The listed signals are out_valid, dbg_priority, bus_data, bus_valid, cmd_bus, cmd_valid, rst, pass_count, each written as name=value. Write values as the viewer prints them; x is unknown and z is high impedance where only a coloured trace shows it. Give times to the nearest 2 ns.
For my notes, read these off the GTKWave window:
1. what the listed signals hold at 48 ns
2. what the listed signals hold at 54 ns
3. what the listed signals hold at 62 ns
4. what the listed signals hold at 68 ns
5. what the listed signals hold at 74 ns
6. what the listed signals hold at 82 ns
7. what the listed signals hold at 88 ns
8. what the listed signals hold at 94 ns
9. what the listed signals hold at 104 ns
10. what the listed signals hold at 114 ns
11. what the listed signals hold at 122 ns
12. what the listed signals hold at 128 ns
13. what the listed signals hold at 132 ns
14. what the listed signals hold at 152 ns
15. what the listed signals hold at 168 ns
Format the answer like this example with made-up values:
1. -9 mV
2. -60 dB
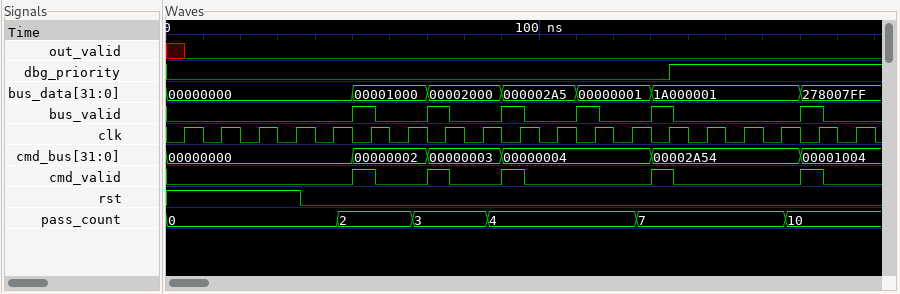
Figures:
1. out_valid=0, dbg_priority=0, bus_data=00000000, bus_valid=0, cmd_bus=00000000, cmd_valid=0, rst=0, pass_count=2
2. out_valid=0, dbg_priority=0, bus_data=00001000, bus_valid=1, cmd_bus=00000002, cmd_valid=1, rst=0, pass_count=2
3. out_valid=0, dbg_priority=0, bus_data=00001000, bus_valid=0, cmd_bus=00000002, cmd_valid=0, rst=0, pass_count=2
4. out_valid=0, dbg_priority=0, bus_data=00001000, bus_valid=0, cmd_bus=00000002, cmd_valid=0, rst=0, pass_count=3
5. out_valid=0, dbg_priority=0, bus_data=00002000, bus_valid=1, cmd_bus=00000003, cmd_valid=1, rst=0, pass_count=3
6. out_valid=0, dbg_priority=0, bus_data=00002000, bus_valid=0, cmd_bus=00000003, cmd_valid=0, rst=0, pass_count=3
7. out_valid=0, dbg_priority=0, bus_data=00002000, bus_valid=0, cmd_bus=00000003, cmd_valid=0, rst=0, pass_count=4
8. out_valid=0, dbg_priority=0, bus_data=000002A5, bus_valid=1, cmd_bus=00000004, cmd_valid=1, rst=0, pass_count=4
9. out_valid=0, dbg_priority=0, bus_data=000002A5, bus_valid=0, cmd_bus=00000004, cmd_valid=0, rst=0, pass_count=4
10. out_valid=0, dbg_priority=0, bus_data=00000001, bus_valid=1, cmd_bus=00000004, cmd_valid=0, rst=0, pass_count=4
11. out_valid=0, dbg_priority=0, bus_data=00000001, bus_valid=0, cmd_bus=00000004, cmd_valid=0, rst=0, pass_count=4
12. out_valid=0, dbg_priority=0, bus_data=00000001, bus_valid=0, cmd_bus=00000004, cmd_valid=0, rst=0, pass_count=7
13. out_valid=0, dbg_priority=0, bus_data=1A000001, bus_valid=1, cmd_bus=00002A54, cmd_valid=1, rst=0, pass_count=7
14. out_valid=0, dbg_priority=1, bus_data=1A000001, bus_valid=0, cmd_bus=00002A54, cmd_valid=0, rst=0, pass_count=7
15. out_valid=0, dbg_priority=1, bus_data=1A000001, bus_valid=0, cmd_bus=00002A54, cmd_valid=0, rst=0, pass_count=10
